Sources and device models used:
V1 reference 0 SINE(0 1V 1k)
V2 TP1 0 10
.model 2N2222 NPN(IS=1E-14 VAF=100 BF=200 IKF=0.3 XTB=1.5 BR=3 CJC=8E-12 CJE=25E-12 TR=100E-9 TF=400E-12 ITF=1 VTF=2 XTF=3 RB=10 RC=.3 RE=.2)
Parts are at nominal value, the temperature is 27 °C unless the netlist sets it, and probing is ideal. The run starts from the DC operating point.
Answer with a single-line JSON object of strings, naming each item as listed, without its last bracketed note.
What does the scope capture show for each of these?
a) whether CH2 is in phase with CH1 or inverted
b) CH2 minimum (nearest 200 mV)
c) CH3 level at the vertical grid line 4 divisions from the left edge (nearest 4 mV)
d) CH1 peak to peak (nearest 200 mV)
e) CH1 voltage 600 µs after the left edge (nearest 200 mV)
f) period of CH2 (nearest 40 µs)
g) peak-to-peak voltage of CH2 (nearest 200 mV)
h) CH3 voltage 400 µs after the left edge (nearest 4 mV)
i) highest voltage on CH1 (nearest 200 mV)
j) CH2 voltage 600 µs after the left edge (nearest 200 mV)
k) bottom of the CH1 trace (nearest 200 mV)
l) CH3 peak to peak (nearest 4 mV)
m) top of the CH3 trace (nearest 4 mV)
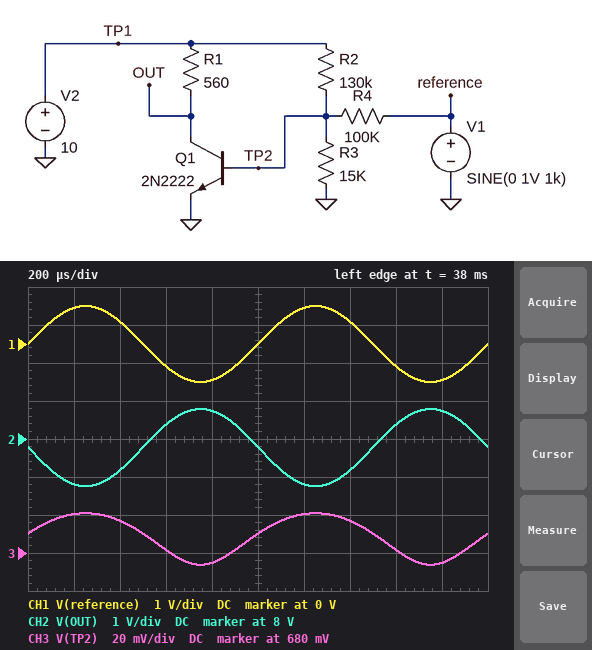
{"whether CH2 is in phase with CH1 or inverted": "inverted", "CH2 minimum": "6.8 V", "CH3 level at the vertical grid line 4 divisions from the left edge": "676 mV", "CH1 peak to peak": "2.0 V", "CH1 voltage 600 µs after the left edge": "-600 mV", "period of CH2": "1.00 ms", "peak-to-peak voltage of CH2": "2.0 V", "CH3 voltage 400 µs after the left edge": "696 mV", "highest voltage on CH1": "1.0 V", "CH2 voltage 600 µs after the left edge": "8.4 V", "bottom of the CH1 trace": "-1.0 V", "CH3 peak to peak": "28 mV", "top of the CH3 trace": "700 mV"}
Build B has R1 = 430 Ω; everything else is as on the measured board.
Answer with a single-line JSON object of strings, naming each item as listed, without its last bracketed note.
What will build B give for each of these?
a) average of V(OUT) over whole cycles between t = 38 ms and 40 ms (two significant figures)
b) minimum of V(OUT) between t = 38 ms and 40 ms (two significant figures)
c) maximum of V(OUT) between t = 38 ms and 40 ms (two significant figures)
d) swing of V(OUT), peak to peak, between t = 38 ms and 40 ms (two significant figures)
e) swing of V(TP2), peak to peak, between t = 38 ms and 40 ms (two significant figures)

{"average of V(OUT) over whole cycles between t = 38 ms and 40 ms": "8.3 V", "minimum of V(OUT) between t = 38 ms and 40 ms": "7.5 V", "maximum of V(OUT) between t = 38 ms and 40 ms": "9.1 V", "swing of V(OUT), peak to peak, between t = 38 ms and 40 ms": "1.6 V", "swing of V(TP2), peak to peak, between t = 38 ms and 40 ms": "27 mV"}
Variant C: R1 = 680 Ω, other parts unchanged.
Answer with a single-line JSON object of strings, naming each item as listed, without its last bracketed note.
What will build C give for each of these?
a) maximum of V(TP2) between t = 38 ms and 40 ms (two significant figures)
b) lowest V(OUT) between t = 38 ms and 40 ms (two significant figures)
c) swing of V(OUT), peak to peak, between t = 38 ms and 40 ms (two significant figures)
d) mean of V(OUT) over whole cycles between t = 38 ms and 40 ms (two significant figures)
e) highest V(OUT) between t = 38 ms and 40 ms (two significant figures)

{"maximum of V(TP2) between t = 38 ms and 40 ms": "700 mV", "lowest V(OUT) between t = 38 ms and 40 ms": "6.1 V", "swing of V(OUT), peak to peak, between t = 38 ms and 40 ms": "2.4 V", "mean of V(OUT) over whole cycles between t = 38 ms and 40 ms": "7.3 V", "highest V(OUT) between t = 38 ms and 40 ms": "8.5 V"}
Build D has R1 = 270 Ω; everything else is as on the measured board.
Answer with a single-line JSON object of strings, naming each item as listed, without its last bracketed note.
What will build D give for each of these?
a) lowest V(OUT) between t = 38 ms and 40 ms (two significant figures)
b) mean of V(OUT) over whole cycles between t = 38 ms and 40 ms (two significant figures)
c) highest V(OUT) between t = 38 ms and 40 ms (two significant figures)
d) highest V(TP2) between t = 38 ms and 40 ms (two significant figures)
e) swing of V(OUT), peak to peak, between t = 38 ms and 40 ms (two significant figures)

{"lowest V(OUT) between t = 38 ms and 40 ms": "8.4 V", "mean of V(OUT) over whole cycles between t = 38 ms and 40 ms": "8.9 V", "highest V(OUT) between t = 38 ms and 40 ms": "9.4 V", "highest V(TP2) between t = 38 ms and 40 ms": "700 mV", "swing of V(OUT), peak to peak, between t = 38 ms and 40 ms": "1.0 V"}
